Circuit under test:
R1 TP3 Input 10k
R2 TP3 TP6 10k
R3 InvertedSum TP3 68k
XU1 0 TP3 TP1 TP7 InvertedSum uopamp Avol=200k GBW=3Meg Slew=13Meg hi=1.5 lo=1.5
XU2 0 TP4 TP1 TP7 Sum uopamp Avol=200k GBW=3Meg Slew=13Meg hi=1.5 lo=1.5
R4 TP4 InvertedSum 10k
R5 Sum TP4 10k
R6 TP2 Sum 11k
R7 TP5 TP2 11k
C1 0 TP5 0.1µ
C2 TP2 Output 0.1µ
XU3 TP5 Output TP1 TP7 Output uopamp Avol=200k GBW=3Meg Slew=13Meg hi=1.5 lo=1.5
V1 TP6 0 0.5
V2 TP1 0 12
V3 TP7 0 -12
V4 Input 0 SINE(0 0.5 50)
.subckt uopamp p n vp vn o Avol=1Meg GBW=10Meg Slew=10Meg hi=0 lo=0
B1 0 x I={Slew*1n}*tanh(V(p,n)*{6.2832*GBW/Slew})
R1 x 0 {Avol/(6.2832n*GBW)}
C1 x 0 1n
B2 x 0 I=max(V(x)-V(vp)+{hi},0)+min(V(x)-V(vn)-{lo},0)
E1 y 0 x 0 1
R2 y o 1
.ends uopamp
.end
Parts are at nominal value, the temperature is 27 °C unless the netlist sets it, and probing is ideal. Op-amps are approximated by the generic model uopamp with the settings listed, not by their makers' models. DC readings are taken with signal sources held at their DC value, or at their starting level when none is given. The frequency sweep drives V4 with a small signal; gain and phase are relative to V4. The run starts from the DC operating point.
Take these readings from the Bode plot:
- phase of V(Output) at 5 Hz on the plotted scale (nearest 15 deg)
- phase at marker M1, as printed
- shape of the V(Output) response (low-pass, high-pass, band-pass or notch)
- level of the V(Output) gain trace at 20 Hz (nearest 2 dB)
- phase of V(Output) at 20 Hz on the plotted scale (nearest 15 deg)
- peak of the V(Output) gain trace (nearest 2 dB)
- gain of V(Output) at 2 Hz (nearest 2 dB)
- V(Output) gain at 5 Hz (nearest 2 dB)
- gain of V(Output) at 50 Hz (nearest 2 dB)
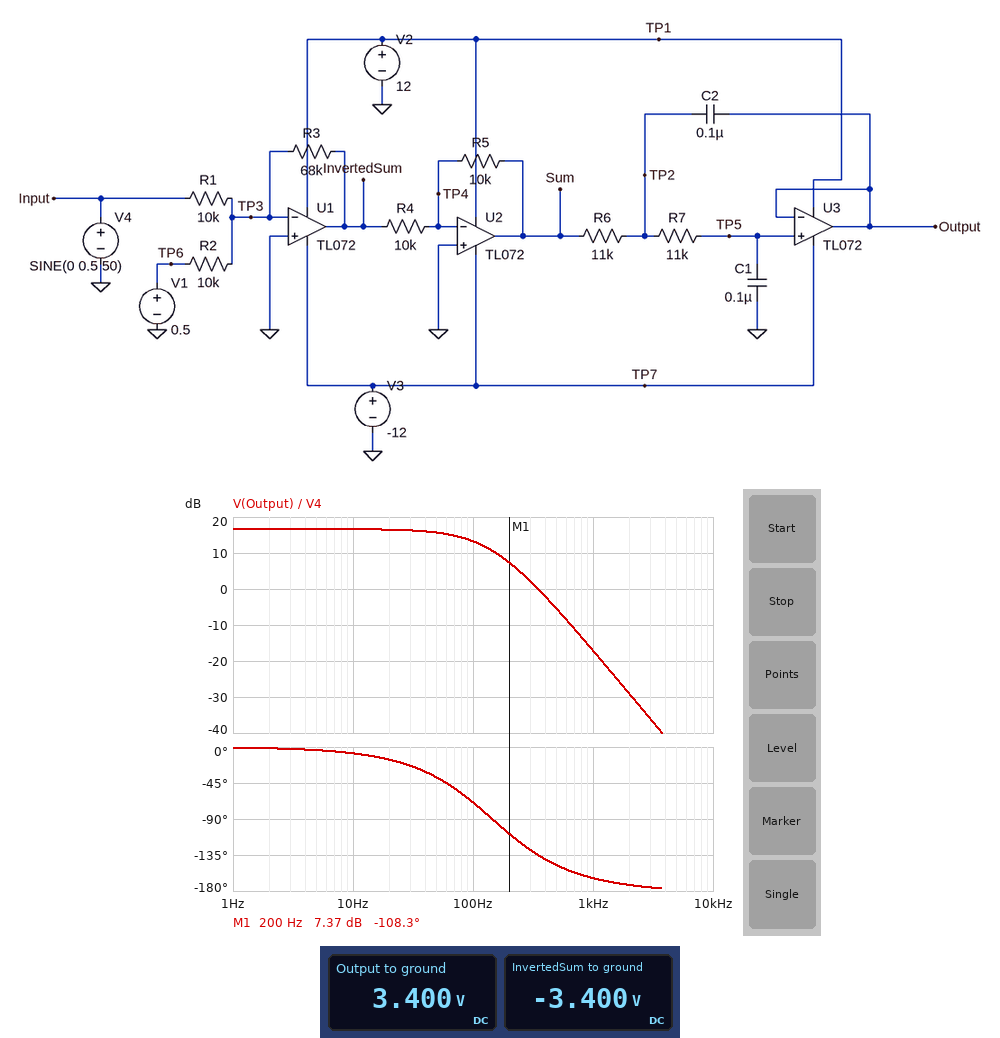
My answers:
0 deg
-108.3 deg
low-pass
16 dB
-15 deg
16 dB
16 dB
16 dB
16 dB
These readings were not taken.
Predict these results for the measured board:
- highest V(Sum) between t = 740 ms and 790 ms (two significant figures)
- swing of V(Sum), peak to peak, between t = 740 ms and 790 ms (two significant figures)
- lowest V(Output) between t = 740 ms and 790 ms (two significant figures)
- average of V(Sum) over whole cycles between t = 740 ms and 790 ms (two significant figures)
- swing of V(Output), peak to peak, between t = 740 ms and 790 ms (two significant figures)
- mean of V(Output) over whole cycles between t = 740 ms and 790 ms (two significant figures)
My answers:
6.8 V
6.8 V
360 mV
3.4 V
6.1 V
3.4 V
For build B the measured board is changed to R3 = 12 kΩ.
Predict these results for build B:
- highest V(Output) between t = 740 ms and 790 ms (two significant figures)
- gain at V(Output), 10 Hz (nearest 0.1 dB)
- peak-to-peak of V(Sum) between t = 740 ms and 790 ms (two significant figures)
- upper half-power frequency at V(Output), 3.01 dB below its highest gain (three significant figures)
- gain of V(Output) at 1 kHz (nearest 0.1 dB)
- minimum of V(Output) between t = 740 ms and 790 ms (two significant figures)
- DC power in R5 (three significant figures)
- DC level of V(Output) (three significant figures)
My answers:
1.1 V
1.5 dB
1.2 V
93.1 Hz
-32.2 dB
64 mV
36.0 µW
600 mV
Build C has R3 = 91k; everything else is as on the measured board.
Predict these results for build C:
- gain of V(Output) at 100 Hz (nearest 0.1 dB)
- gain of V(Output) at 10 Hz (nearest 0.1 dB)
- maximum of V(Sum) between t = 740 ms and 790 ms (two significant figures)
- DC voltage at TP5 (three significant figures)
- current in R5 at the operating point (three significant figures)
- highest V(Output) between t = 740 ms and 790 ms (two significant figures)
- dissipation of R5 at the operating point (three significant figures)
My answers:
15.8 dB
19.1 dB
9.1 V
4.55 V
455 µA
8.6 V
2.07 mW
